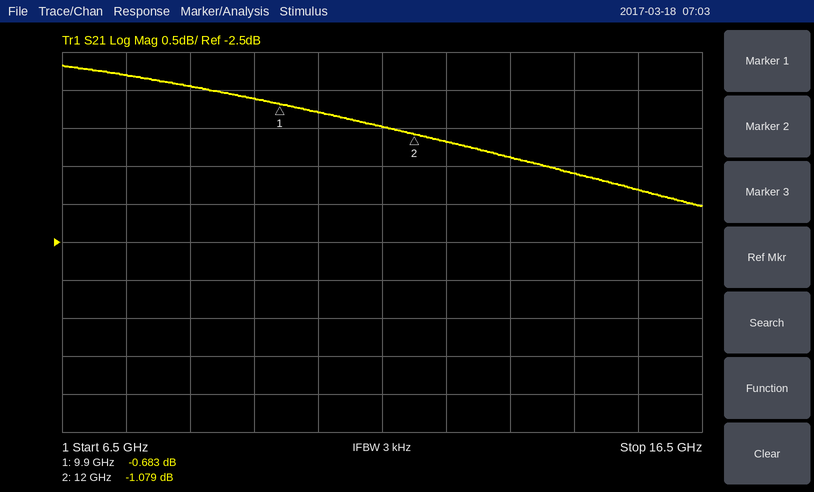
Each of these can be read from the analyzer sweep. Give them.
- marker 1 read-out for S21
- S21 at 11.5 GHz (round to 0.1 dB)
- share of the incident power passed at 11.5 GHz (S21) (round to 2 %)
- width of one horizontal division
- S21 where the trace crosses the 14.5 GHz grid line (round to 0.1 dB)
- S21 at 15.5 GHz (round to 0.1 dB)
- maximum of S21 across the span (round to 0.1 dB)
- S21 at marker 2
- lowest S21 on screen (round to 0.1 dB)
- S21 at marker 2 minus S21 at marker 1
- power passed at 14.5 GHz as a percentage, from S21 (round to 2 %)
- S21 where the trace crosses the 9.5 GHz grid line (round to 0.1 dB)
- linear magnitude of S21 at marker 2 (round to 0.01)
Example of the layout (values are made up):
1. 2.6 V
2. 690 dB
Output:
1. -0.683 dB
2. -1.0 dB
3. 80 %
4. 1 GHz
5. -1.6 dB
6. -1.8 dB
7. -0.2 dB
8. -1.079 dB
9. -2.0 dB
10. -0.396 dB
11. 70 %
12. -0.6 dB
13. 0.88
